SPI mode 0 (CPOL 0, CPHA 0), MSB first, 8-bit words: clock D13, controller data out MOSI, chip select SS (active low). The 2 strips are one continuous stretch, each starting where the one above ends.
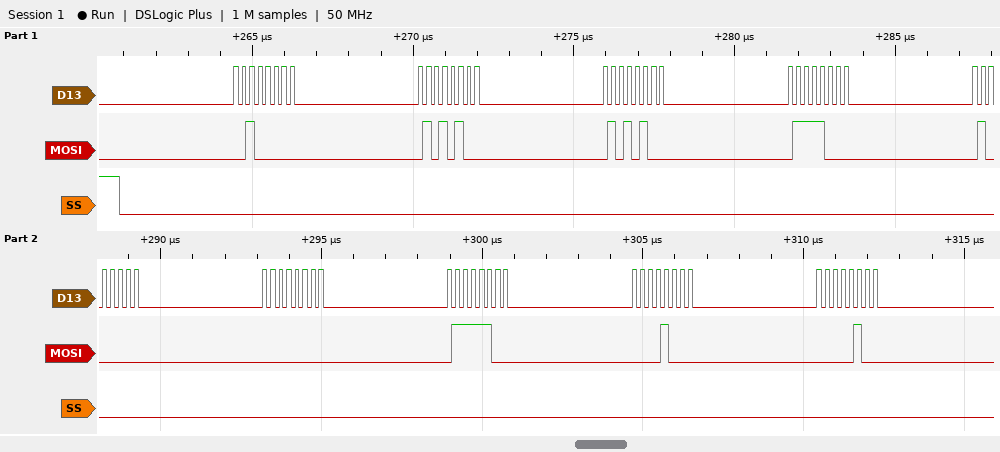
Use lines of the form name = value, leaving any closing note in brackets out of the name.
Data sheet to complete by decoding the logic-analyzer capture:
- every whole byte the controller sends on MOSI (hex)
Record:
every whole byte the controller sends on MOSI = 20 54 54 78 40 00 7C 08 04
